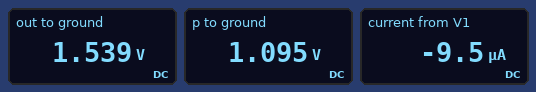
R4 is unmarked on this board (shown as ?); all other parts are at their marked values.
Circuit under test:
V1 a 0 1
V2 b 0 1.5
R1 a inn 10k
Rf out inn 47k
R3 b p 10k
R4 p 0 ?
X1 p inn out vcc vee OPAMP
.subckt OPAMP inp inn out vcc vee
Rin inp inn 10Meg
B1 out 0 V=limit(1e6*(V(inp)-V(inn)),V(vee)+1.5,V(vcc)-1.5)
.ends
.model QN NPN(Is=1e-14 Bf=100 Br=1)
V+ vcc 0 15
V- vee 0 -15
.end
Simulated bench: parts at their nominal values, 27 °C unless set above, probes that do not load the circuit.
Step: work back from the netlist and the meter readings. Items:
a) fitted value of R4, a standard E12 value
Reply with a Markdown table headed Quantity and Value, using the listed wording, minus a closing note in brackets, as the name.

| Quantity | Value |
|---|---|
| fitted value of R4, a standard E12 value | 27 kΩ |
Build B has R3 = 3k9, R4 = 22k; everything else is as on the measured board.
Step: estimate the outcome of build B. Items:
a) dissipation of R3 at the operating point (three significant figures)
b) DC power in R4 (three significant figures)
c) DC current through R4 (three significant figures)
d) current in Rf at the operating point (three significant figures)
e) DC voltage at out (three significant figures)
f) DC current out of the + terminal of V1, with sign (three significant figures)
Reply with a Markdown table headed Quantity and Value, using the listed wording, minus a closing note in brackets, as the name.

| Quantity | Value |
|---|---|
| dissipation of R3 at the operating point | 13.1 µW |
| DC power in R4 | 73.8 µW |
| DC current through R4 | 57.9 µA |
| current in Rf at the operating point | 27.4 µA |
| DC voltage at out | 2.56 V |
| DC current out of the + terminal of V1, with sign | -27.4 µA |
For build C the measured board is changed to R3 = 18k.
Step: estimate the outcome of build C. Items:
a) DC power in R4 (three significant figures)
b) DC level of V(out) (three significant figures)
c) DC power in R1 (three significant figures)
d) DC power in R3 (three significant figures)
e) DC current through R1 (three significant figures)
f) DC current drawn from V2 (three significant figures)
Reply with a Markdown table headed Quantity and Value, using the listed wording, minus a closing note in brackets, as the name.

| Quantity | Value |
|---|---|
| DC power in R4 | 30.0 µW |
| DC level of V(out) | 430 mV |
| DC power in R1 | 1.00 µW |
| DC power in R3 | 20.0 µW |
| DC current through R1 | 10.0 µA |
| DC current drawn from V2 | 33.3 µA |
